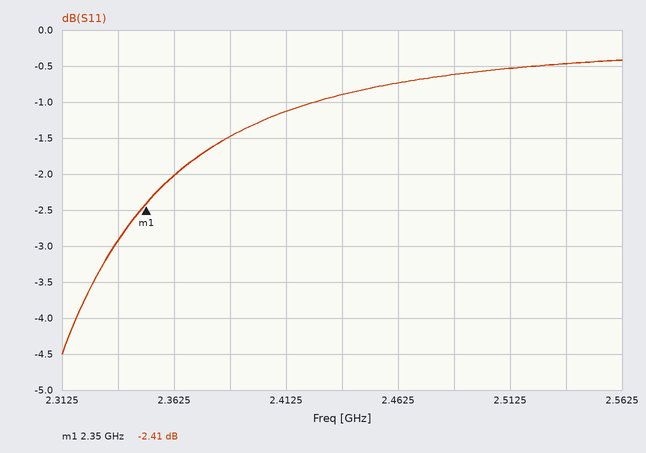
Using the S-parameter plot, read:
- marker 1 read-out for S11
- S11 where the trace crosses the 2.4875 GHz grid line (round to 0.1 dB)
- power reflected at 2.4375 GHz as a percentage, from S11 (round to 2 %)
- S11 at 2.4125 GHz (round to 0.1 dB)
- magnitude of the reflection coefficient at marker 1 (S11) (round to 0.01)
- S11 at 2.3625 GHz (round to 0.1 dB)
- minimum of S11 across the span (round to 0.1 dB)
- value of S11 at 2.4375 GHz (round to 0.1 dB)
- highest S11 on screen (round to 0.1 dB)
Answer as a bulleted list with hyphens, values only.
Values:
- -2.41 dB
- -0.6 dB
- 82 %
- -1.1 dB
- 0.76
- -2.0 dB
- -4.5 dB
- -0.9 dB
- -0.4 dB
